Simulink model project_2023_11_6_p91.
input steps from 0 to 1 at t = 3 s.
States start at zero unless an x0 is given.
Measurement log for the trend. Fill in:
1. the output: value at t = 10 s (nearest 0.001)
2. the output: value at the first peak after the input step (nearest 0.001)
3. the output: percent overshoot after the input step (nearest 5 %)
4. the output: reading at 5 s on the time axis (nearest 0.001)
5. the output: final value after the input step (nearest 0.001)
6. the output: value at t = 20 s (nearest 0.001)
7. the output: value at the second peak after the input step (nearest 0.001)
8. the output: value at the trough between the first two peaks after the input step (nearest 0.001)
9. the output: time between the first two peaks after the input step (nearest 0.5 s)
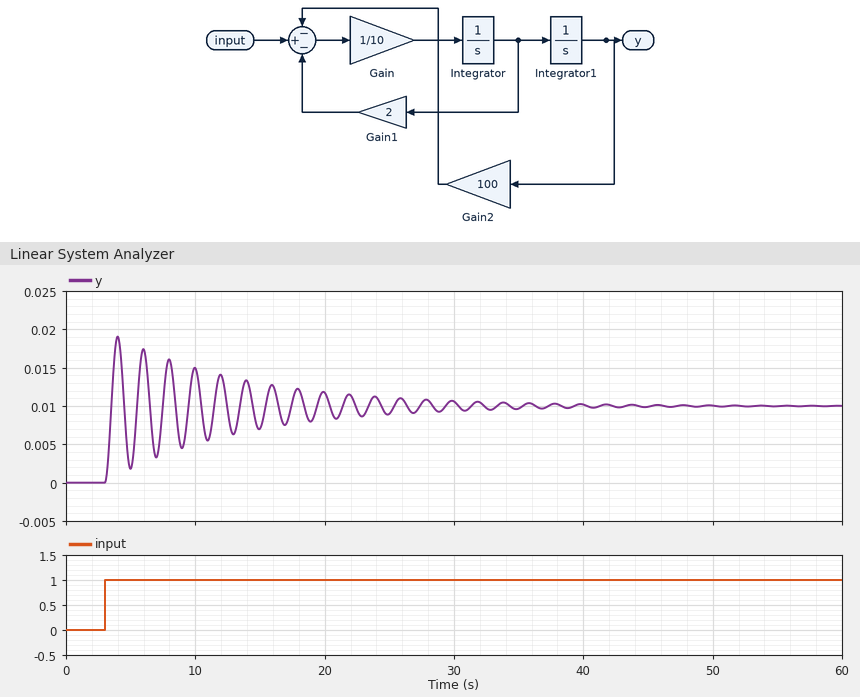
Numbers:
0.015
0.019
90 %
0.002
0.010
0.012
0.017
0.002
2.0 s
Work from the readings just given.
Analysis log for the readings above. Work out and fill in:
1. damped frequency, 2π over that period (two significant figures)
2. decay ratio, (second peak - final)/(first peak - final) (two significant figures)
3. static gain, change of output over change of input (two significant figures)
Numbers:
3.1 rad/s
0.78
0.010
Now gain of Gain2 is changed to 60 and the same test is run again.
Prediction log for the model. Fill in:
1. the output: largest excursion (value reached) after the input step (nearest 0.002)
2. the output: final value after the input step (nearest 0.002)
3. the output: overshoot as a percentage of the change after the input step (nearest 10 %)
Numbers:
0.032
0.016
90 %
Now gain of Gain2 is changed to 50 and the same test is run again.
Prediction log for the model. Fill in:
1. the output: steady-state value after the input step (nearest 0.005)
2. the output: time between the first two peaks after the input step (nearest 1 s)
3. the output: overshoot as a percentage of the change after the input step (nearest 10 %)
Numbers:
0.020
3 s
90 %
